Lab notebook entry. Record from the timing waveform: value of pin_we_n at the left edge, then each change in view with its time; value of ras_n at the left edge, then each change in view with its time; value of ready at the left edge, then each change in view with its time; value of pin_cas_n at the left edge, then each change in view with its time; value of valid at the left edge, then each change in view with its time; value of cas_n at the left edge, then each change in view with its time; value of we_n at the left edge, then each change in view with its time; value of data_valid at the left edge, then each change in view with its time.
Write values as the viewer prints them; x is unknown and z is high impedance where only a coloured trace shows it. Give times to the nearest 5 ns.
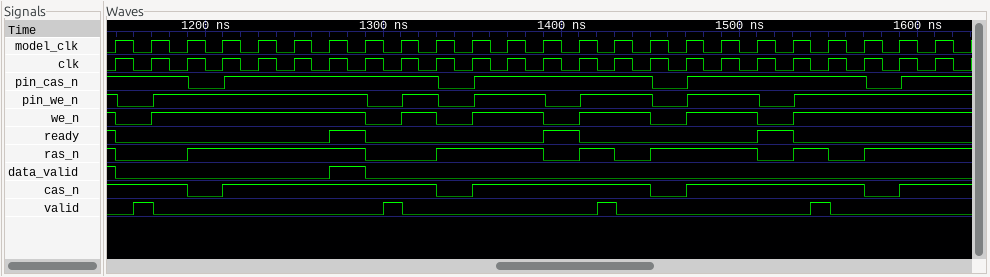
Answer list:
1, 0 at 1150 ns, 1 at 1170 ns, 0 at 1290 ns, 1 at 1310 ns, 0 at 1330 ns, 1 at 1350 ns, 0 at 1390 ns, 1 at 1410 ns, 0 at 1450 ns, 1 at 1470 ns, 0 at 1510 ns, 1 at 1530 ns
1, 0 at 1150 ns, 1 at 1190 ns, 0 at 1290 ns, 1 at 1330 ns, 0 at 1390 ns, 1 at 1410 ns, 0 at 1430 ns, 1 at 1450 ns, 0 at 1510 ns, 1 at 1530 ns, 0 at 1550 ns, 1 at 1570 ns
1, 0 at 1150 ns, 1 at 1270 ns, 0 at 1290 ns, 1 at 1390 ns, 0 at 1410 ns, 1 at 1510 ns, 0 at 1530 ns
1, 0 at 1190 ns, 1 at 1210 ns, 0 at 1330 ns, 1 at 1350 ns, 0 at 1450 ns, 1 at 1470 ns, 0 at 1570 ns, 1 at 1590 ns
0, 1 at 1160 ns, 0 at 1170 ns, 1 at 1300 ns, 0 at 1310 ns, 1 at 1420 ns, 0 at 1430 ns, 1 at 1540 ns, 0 at 1550 ns
1, 0 at 1190 ns, 1 at 1210 ns, 0 at 1330 ns, 1 at 1350 ns, 0 at 1450 ns, 1 at 1470 ns, 0 at 1570 ns, 1 at 1590 ns
1, 0 at 1150 ns, 1 at 1170 ns, 0 at 1290 ns, 1 at 1310 ns, 0 at 1330 ns, 1 at 1350 ns, 0 at 1390 ns, 1 at 1410 ns, 0 at 1450 ns, 1 at 1470 ns, 0 at 1510 ns, 1 at 1530 ns
1, 0 at 1150 ns, 1 at 1270 ns, 0 at 1290 ns
